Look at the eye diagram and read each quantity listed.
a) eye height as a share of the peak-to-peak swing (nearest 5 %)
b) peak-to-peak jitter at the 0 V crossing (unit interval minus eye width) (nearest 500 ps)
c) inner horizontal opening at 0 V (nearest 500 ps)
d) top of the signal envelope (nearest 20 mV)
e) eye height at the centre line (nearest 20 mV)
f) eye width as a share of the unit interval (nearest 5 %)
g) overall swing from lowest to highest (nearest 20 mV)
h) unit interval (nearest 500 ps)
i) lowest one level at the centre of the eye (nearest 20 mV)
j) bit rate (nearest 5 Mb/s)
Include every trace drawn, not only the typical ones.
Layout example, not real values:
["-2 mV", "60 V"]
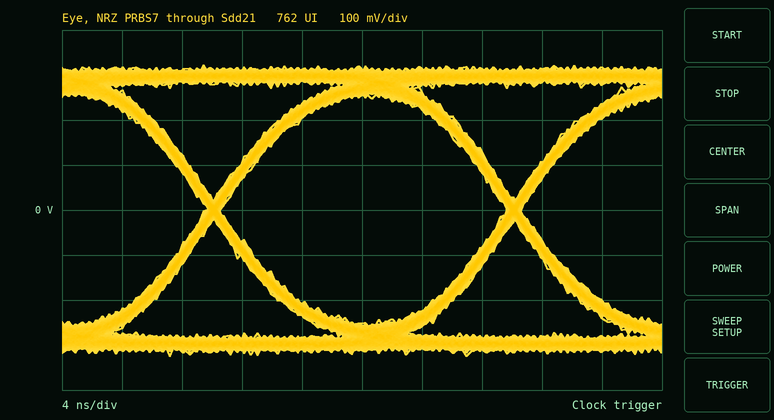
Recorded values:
["80 %", "1.0 ns", "19.0 ns", "320 mV", "500 mV", "95 %", "640 mV", "20.0 ns", "260 mV", "50 Mb/s"]
